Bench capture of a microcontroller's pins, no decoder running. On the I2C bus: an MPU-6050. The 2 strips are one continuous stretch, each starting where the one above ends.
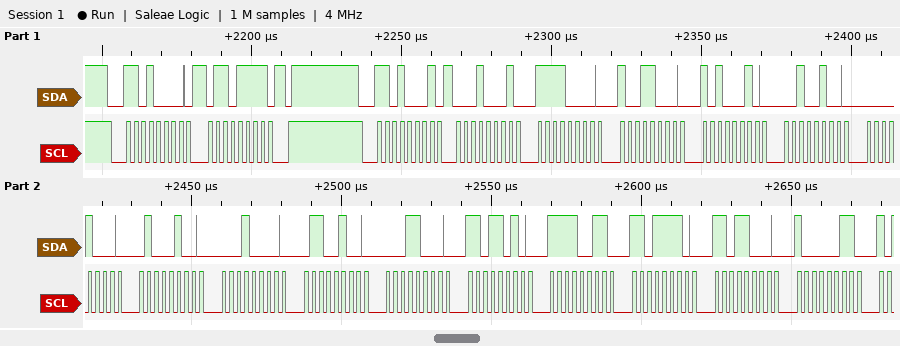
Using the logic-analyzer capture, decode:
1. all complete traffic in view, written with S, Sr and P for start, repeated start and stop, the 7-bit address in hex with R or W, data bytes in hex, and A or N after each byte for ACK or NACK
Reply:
S 68W A 6F A P S 68R A 11 A F0 A 98 A A2 A 24 A 08 A 44 A 10 A 64 A 18 A DA A F3 A DE A D8 A 83 A
